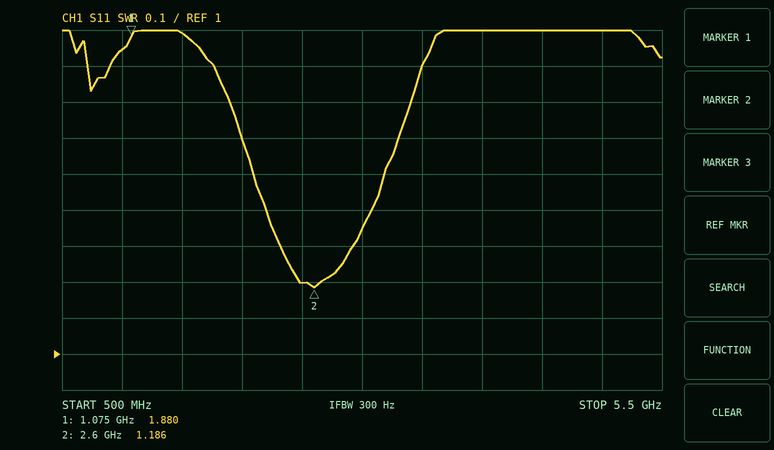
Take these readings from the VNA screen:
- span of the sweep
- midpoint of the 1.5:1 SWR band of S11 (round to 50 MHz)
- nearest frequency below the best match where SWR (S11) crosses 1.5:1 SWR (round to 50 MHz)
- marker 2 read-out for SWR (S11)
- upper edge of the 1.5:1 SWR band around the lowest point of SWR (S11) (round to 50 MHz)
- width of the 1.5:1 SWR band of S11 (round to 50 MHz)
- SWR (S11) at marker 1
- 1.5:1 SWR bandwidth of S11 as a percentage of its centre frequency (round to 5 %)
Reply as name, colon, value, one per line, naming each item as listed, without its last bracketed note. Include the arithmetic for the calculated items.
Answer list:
span of the sweep: 5 GHz
midpoint of the 1.5:1 SWR band of S11: 2.65 GHz
nearest frequency below the best match where SWR (S11) crosses 1.5:1 SWR: 2.10 GHz
marker 2 read-out for SWR: 1.186
upper edge of the 1.5:1 SWR band around the lowest point of SWR (S11): 3.20 GHz
width of the 1.5:1 SWR band of S11: 3.20 GHz − 2.10 GHz = 1.10 GHz
SWR (S11) at marker 1: 1.880
1.5:1 SWR bandwidth of S11 as a percentage of its centre frequency: 1.1 GHz / 2.65 GHz ≈ 41.5 %, so 40 % to the nearest 5 %
